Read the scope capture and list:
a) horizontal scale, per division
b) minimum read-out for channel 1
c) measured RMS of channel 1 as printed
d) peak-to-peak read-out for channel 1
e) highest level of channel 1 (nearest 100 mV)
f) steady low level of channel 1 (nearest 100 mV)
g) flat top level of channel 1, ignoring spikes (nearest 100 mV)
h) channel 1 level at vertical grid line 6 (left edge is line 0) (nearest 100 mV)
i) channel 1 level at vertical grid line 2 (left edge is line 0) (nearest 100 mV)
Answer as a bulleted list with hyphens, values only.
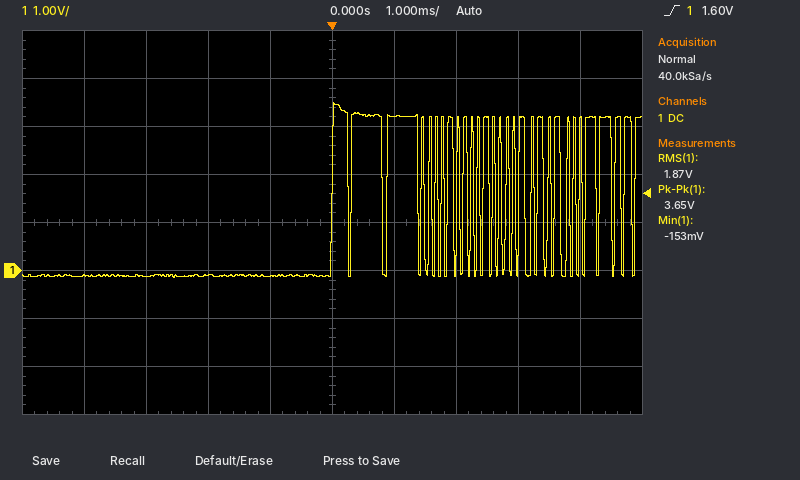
- 1 ms
- -153 mV
- 1.87 V
- 3.65 V
- 3.5 V
- -100 mV
- 3.2 V
- 3.2 V
- -100 mV
